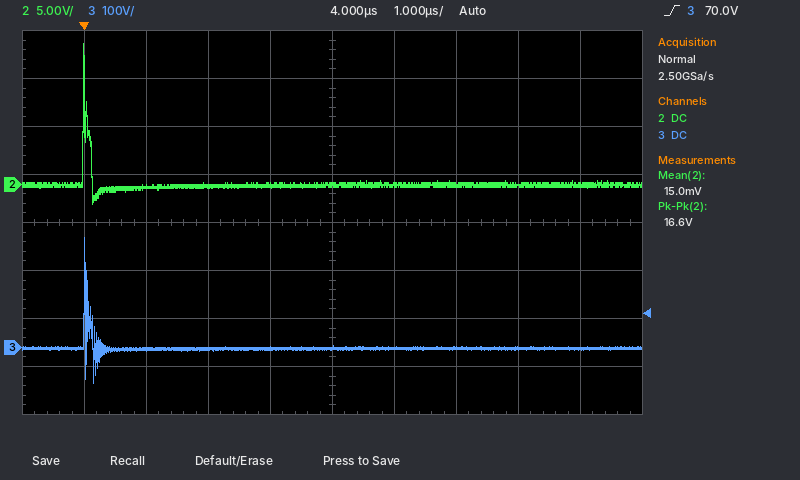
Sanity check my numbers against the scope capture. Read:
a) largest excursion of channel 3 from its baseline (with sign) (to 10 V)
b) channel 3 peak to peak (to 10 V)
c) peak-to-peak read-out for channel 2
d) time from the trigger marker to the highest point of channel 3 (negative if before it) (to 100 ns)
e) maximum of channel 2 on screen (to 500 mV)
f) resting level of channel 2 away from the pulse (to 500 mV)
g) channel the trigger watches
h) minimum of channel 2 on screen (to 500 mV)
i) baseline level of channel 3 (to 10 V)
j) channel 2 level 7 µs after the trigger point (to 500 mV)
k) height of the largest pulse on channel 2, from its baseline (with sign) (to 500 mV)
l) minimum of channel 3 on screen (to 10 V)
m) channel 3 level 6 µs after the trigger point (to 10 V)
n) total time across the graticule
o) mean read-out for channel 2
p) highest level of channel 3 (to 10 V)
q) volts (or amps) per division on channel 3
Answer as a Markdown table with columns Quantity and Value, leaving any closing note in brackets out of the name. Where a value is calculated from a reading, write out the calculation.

| Quantity | Value |
|---|---|
| largest excursion of channel 3 from its baseline (with sign) | 230 V − (0 V) = +230 V |
| channel 3 peak to peak | 230 V − (-70 V) = 300 V |
| peak-to-peak read-out for channel 2 | 16.6 V |
| time from the trigger marker to the highest point of channel 3 (negative if before it) | 0.0 µs |
| maximum of channel 2 on screen | 14.5 V |
| resting level of channel 2 away from the pulse | 0.0 V |
| channel the trigger watches | channel 3 |
| minimum of channel 2 on screen | -2.0 V |
| baseline level of channel 3 | 0 V |
| channel 2 level 7 µs after the trigger point | 0.0 V |
| height of the largest pulse on channel 2, from its baseline (with sign) | 14.5 V − (0.0 V) = +14.5 V |
| minimum of channel 3 on screen | -70 V |
| channel 3 level 6 µs after the trigger point | 0 V |
| total time across the graticule | 10 µs |
| mean read-out for channel 2 | 15.0 mV |
| highest level of channel 3 | 230 V |
| volts (or amps) per division on channel 3 | 100 V |
